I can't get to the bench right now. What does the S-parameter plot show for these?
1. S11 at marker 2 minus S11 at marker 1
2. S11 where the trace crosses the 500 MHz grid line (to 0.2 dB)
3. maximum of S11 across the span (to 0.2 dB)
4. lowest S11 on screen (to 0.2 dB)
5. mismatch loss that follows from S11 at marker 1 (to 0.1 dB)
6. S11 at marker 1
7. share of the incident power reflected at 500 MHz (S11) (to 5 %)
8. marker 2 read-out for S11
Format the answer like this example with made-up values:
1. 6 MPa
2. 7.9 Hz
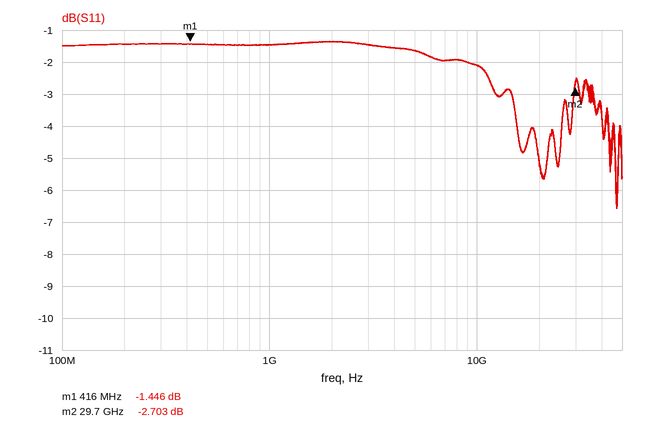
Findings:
1. -1.257 dB
2. -1.4 dB
3. -1.4 dB
4. -6.6 dB
5. 5.5 dB
6. -1.446 dB
7. 70 %
8. -2.703 dB
